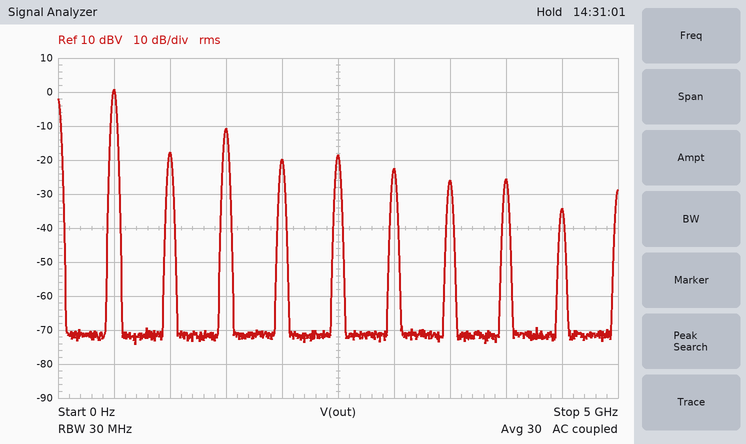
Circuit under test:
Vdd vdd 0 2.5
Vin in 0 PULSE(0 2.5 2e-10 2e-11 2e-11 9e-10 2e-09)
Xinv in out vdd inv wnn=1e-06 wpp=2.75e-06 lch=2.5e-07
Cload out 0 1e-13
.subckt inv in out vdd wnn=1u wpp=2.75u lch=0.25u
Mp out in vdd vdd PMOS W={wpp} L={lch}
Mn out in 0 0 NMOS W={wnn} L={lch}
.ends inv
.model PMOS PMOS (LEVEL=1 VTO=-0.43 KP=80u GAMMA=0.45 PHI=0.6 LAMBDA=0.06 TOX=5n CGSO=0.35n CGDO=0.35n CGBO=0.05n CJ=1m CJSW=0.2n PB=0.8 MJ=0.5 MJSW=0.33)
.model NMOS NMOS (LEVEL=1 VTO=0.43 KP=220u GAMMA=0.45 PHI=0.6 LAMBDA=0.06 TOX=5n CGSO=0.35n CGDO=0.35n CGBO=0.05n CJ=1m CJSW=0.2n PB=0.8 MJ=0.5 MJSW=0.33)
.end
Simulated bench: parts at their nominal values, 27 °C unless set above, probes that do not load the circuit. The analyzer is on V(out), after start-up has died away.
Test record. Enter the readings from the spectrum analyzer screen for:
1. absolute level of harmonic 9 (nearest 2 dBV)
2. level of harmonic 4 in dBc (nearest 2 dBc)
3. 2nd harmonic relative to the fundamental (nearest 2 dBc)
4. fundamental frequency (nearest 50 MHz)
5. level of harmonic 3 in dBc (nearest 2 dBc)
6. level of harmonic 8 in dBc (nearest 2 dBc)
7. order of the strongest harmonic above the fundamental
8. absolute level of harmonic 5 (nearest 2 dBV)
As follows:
-34 dBV
-20 dBc
-18 dBc
500 MHz
-12 dBc
-26 dBc
3
-18 dBV
